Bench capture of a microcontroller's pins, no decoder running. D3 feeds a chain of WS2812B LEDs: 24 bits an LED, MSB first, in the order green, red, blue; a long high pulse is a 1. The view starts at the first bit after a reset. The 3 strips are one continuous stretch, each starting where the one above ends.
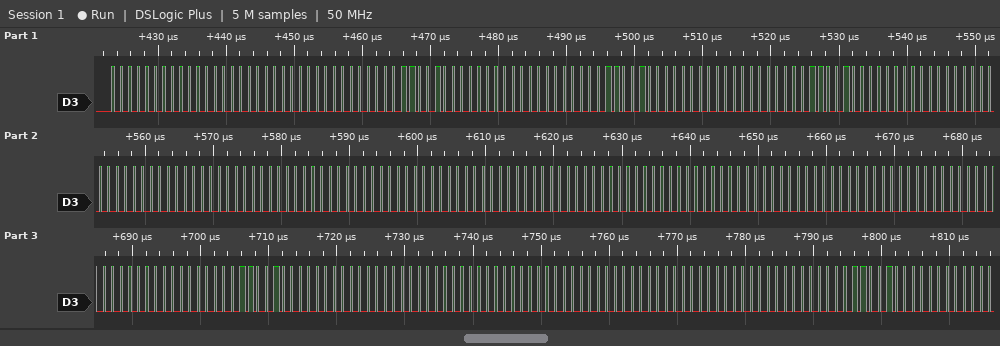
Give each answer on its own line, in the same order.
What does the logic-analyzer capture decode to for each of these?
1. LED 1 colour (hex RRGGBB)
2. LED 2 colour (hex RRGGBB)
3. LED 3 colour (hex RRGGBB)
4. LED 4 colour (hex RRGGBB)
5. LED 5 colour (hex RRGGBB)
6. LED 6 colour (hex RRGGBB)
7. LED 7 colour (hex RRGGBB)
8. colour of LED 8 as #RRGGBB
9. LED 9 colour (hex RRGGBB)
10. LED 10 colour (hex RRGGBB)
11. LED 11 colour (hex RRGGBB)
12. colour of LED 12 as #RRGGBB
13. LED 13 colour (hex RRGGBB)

#000000
#320000
#320000
#320000
#000000
#000000
#000000
#000000
#000000
#320000
#000000
#000000
#320000
